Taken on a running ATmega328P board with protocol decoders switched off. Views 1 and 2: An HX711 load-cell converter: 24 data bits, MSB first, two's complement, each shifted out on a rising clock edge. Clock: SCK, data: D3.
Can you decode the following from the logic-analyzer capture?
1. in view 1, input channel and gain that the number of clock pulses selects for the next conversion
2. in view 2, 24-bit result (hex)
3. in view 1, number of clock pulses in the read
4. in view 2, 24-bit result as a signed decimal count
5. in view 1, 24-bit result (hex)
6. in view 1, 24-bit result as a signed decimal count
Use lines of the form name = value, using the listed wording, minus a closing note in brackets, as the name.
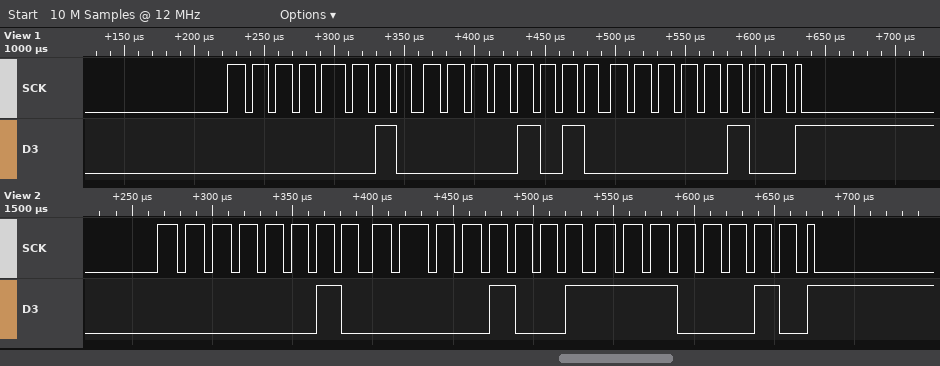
in view 1, input channel and gain that the number of clock pulses selects for the next conversion = channel A, gain 128
in view 2, 24-bit result = 0x0209E2
in view 1, number of clock pulses in the read = 25
in view 2, 24-bit result as a signed decimal count = 133602
in view 1, 24-bit result = 0x020A04
in view 1, 24-bit result as a signed decimal count = 133636
